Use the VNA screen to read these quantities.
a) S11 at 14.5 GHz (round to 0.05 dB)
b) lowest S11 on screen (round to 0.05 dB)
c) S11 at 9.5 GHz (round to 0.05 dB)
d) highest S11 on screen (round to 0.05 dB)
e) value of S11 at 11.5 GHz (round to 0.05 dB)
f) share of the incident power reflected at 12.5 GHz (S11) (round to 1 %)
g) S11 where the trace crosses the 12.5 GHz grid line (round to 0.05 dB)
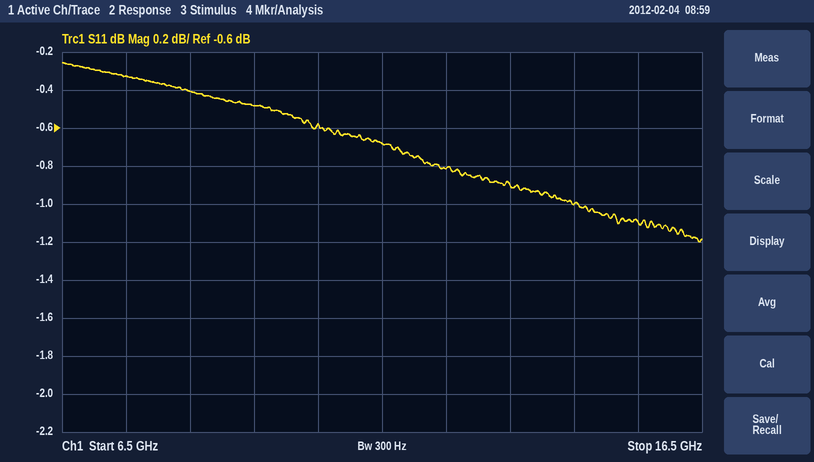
-1.00 dB
-1.20 dB
-0.50 dB
-0.25 dB
-0.70 dB
83 %
-0.80 dB
